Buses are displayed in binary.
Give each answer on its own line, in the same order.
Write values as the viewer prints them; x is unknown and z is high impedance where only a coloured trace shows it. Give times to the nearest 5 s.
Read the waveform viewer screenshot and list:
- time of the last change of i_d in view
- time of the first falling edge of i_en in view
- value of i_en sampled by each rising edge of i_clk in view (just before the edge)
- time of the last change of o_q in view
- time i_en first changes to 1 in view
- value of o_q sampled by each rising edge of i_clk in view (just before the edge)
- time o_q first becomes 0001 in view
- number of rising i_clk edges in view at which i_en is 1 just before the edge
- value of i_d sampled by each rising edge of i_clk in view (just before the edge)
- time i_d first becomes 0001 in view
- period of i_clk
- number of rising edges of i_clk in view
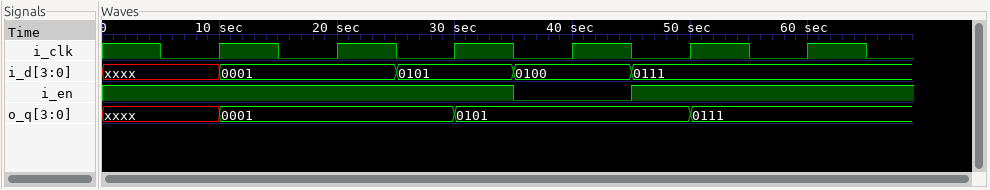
45 s
35 s
1 1 1 0 1 1
50 s
45 s
xxxx, 0001, 0001, 0101, 0101, 0111
10 s
5
xxxx, 0001, 0101, 0100, 0111, 0111
10 s
10 s
6
